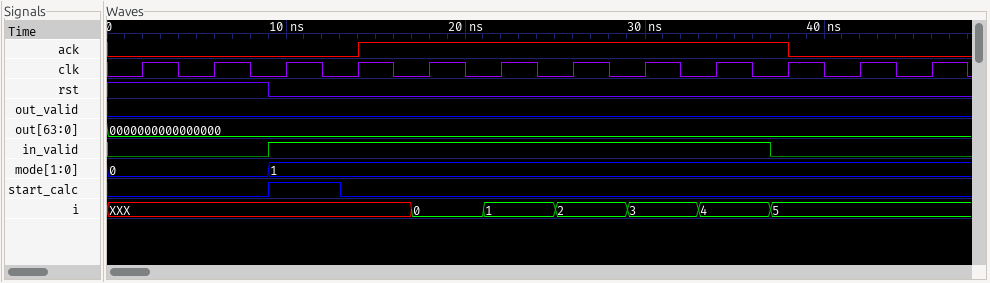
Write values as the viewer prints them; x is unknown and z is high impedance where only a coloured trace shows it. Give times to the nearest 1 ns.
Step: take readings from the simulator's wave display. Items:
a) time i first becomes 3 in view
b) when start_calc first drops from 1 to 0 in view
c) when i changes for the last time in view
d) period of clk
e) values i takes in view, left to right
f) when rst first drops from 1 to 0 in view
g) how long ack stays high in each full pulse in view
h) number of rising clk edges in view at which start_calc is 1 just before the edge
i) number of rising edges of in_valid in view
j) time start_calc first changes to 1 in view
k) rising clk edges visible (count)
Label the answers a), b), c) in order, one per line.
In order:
a) 29 ns
b) 13 ns
c) 37 ns
d) 4 ns
e) XXX, 0, 1, 2, 3, 4, 5
f) 9 ns
g) 24 ns
h) 1
i) 1
j) 9 ns
k) 12
